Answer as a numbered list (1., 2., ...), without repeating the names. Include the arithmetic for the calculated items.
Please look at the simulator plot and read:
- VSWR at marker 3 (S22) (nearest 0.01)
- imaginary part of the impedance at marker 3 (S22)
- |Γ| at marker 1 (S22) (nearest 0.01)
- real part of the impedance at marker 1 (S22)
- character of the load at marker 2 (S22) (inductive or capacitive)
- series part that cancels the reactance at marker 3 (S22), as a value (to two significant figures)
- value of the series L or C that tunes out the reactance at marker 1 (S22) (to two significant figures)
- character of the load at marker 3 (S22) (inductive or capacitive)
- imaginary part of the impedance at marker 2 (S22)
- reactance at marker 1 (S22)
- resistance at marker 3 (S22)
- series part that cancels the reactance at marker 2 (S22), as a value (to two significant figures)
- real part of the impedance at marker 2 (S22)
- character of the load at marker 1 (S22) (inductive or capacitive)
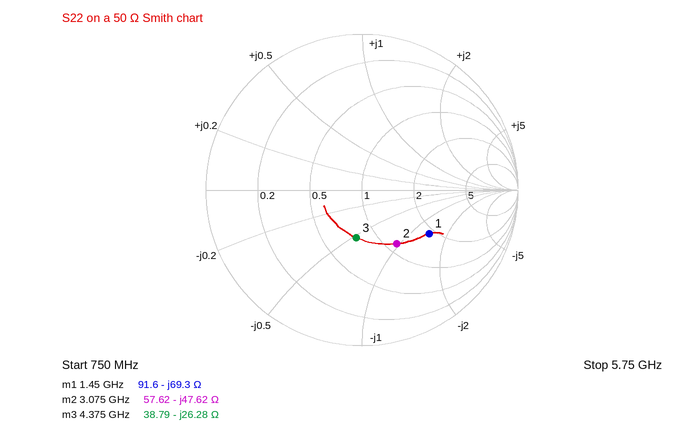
1. 1.89
2. -26.28 Ω
3. 0.51
4. 91.6 Ω
5. capacitive
6. L = 26.28 Ω/(2π × 4.375 GHz) ≈ 956 pH, so 960 pH to two significant figures
7. L = 69.3 Ω/(2π × 1.45 GHz) ≈ 7.6 nH
8. capacitive
9. -47.62 Ω
10. -69.3 Ω
11. 38.79 Ω
12. L = 47.62 Ω/(2π × 3.075 GHz) ≈ 2.5 nH
13. 57.62 Ω
14. capacitive
